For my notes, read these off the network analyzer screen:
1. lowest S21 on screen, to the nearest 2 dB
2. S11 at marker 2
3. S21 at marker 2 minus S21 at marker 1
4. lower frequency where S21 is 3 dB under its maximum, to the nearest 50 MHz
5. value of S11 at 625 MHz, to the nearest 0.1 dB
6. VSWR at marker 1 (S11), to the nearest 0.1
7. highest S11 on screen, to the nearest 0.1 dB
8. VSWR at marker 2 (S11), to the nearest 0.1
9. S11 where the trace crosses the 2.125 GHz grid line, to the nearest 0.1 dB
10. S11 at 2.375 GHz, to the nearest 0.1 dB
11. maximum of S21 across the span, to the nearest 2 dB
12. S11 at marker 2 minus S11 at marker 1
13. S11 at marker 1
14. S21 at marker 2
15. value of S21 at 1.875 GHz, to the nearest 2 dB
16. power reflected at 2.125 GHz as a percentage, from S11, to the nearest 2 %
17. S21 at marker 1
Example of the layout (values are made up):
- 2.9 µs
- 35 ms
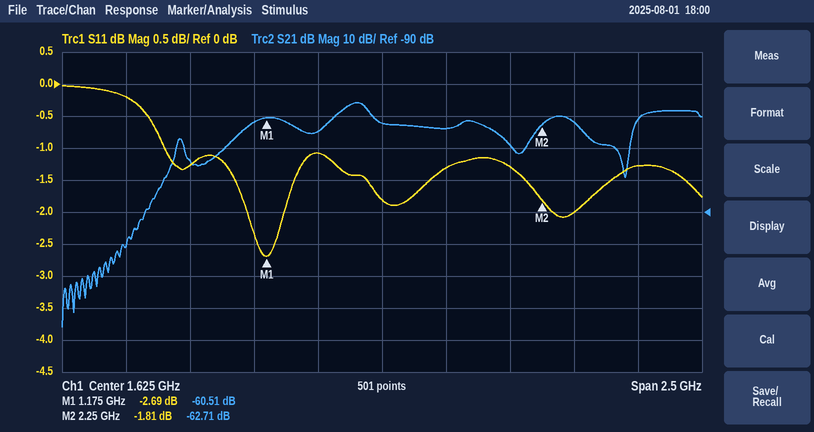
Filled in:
- -126 dB
- -1.81 dB
- -2.20 dB
- 1.45 GHz
- -0.2 dB
- 6.5
- 0.0 dB
- 9.6
- -1.3 dB
- -2.0 dB
- -56 dB
- 0.88 dB
- -2.69 dB
- -62.71 dB
- -64 dB
- 74 %
- -60.51 dB
